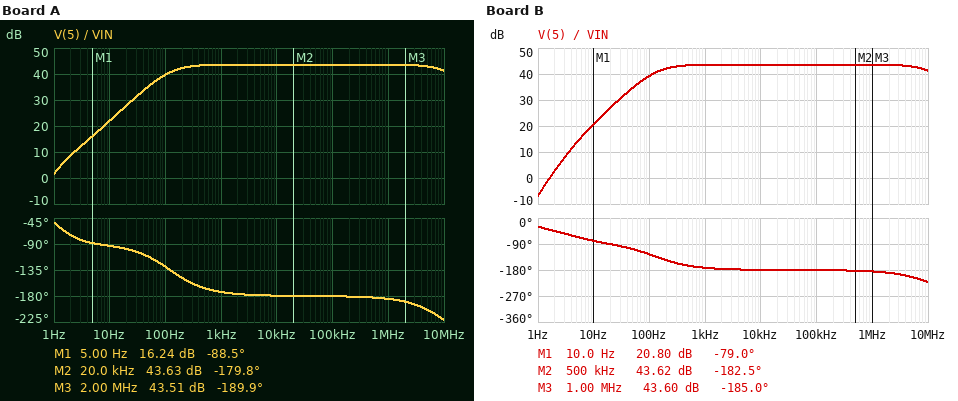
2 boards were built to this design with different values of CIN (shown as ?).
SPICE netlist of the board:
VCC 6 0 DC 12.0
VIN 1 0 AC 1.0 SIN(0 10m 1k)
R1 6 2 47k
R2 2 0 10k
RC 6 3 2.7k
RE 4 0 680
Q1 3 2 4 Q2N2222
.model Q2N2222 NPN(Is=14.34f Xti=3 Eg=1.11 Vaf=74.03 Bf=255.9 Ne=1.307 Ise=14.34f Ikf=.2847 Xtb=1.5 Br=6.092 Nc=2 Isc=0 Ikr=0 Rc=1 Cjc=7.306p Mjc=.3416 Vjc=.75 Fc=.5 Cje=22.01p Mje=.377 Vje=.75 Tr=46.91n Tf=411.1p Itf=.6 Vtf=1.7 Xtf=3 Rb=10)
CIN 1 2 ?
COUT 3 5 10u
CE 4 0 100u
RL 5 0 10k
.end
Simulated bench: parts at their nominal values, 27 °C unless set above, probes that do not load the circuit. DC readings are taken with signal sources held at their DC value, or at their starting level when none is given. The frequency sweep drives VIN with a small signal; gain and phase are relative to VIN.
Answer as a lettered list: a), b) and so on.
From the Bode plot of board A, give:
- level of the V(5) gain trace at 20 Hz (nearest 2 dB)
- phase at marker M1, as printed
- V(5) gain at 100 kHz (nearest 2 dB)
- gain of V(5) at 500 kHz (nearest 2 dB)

a) 28 dB
b) -88.5 deg
c) 44 dB
d) 44 dB
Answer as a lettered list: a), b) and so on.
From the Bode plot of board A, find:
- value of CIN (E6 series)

a) 15 µF
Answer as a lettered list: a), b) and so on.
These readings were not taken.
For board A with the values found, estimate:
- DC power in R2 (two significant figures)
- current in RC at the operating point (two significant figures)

a) 400 µW
b) 2.0 mA
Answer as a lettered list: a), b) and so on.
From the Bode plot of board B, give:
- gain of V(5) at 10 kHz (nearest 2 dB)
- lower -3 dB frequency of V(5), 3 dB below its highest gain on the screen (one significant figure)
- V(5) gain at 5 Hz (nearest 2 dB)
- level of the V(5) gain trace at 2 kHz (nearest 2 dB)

a) 44 dB
b) 100 Hz
c) 14 dB
d) 44 dB
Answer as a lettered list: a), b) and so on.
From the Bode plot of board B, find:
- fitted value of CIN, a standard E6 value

a) 4.7 µF
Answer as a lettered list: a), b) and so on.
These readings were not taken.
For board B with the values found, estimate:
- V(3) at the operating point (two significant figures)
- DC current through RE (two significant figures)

a) 6.7 V
b) 2.0 mA
